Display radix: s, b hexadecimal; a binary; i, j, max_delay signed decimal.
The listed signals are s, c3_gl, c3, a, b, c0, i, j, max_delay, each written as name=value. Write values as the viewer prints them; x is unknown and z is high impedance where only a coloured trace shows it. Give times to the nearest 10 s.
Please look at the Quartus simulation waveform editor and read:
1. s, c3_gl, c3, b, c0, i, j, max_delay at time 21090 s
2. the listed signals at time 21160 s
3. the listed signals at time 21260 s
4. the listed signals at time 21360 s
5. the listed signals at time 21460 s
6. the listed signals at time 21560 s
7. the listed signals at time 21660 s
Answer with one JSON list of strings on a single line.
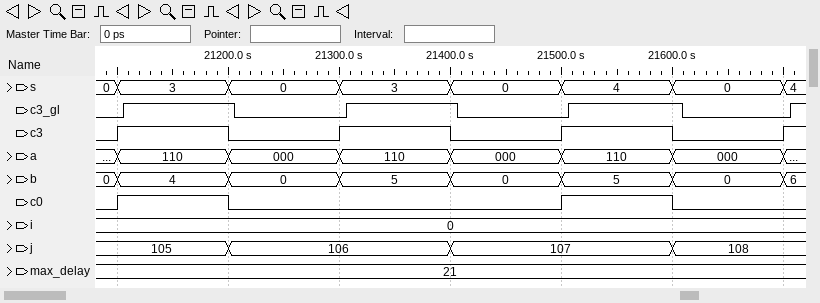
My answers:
["s=0, c3_gl=0, c3=0, b=0, c0=0, i=0, j=105, max_delay=21", "s=3, c3_gl=1, c3=1, a=110, b=4, c0=1, i=0, j=105, max_delay=21", "s=0, c3_gl=0, c3=0, a=000, b=0, c0=0, i=0, j=106, max_delay=21", "s=3, c3_gl=1, c3=1, a=110, b=5, c0=0, i=0, j=106, max_delay=21", "s=0, c3_gl=0, c3=0, a=000, b=0, c0=0, i=0, j=107, max_delay=21", "s=4, c3_gl=1, c3=1, a=110, b=5, c0=1, i=0, j=107, max_delay=21", "s=0, c3_gl=0, c3=0, a=000, b=0, c0=0, i=0, j=108, max_delay=21"]
